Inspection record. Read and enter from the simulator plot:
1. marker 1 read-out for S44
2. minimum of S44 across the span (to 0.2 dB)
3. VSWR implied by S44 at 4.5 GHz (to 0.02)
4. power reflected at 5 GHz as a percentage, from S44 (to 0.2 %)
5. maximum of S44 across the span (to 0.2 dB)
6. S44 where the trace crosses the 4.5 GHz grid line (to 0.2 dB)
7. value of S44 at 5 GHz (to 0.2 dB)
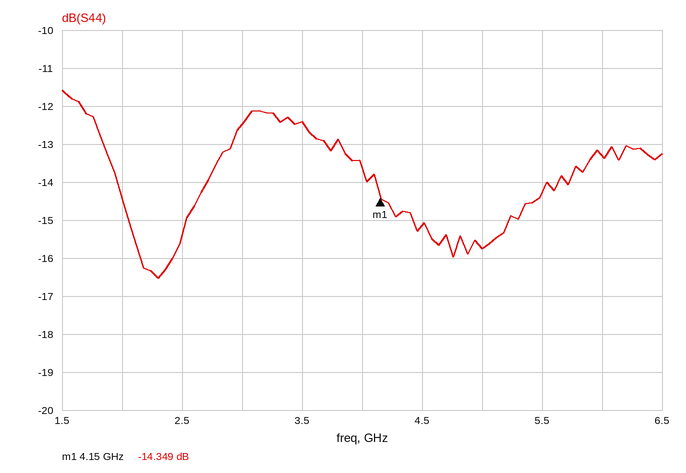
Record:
-14.349 dB
-16.6 dB
1.42
2.6 %
-11.6 dB
-15.2 dB
-15.8 dB
